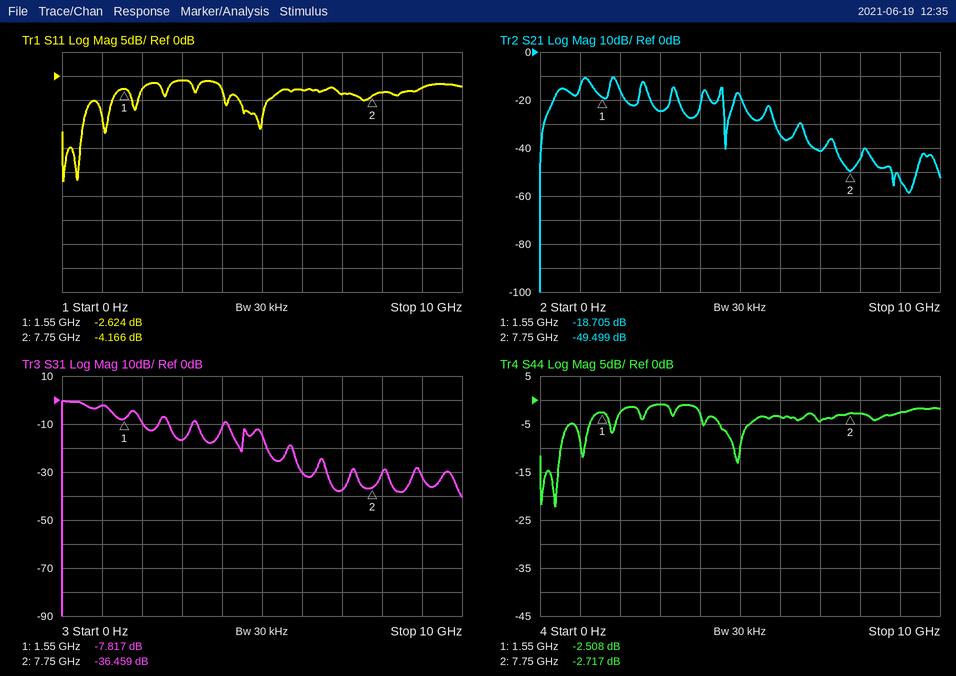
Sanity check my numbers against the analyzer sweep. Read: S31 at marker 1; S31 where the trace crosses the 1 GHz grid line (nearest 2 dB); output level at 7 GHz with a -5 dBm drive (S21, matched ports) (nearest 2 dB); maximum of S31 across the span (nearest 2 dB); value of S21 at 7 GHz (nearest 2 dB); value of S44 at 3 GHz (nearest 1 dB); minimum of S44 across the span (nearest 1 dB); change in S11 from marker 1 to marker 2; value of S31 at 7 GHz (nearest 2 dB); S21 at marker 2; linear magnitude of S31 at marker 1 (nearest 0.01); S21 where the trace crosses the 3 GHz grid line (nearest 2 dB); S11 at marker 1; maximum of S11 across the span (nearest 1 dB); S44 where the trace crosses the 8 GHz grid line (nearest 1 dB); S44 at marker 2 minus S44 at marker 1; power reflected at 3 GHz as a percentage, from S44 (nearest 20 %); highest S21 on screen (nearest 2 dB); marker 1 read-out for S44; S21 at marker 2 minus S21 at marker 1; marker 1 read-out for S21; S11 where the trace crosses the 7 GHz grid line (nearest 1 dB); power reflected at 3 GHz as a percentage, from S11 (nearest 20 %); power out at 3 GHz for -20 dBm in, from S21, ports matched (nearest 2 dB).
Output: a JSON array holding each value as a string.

["-7.817 dB", "-2 dB", "-46 dBm", "0 dB", "-42 dB", "-1 dB", "-22 dB", "-1.542 dB", "-38 dB", "-49.499 dB", "0.41", "-24 dB", "-2.624 dB", "-1 dB", "-3 dB", "-0.209 dB", "80 %", "-10 dB", "-2.508 dB", "-30.794 dB", "-18.705 dB", "-4 dB", "80 %", "-44 dBm"]
